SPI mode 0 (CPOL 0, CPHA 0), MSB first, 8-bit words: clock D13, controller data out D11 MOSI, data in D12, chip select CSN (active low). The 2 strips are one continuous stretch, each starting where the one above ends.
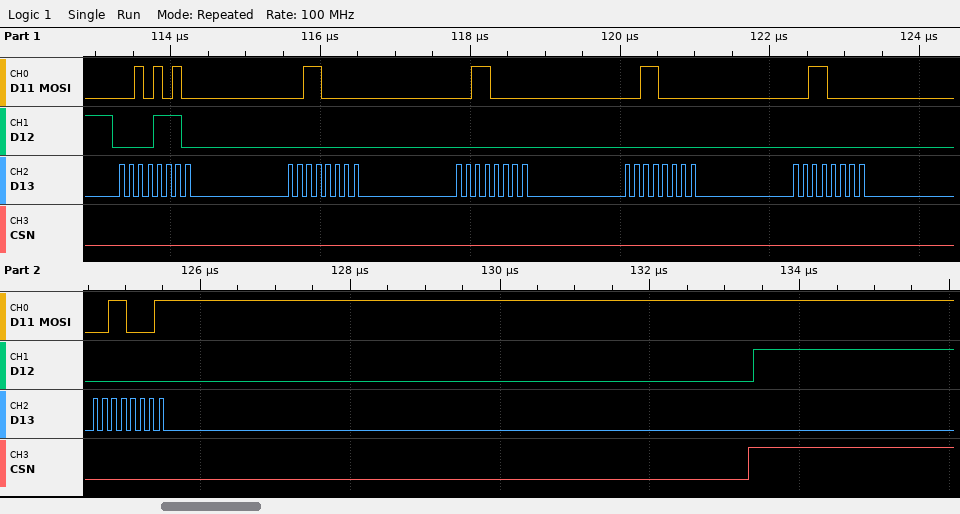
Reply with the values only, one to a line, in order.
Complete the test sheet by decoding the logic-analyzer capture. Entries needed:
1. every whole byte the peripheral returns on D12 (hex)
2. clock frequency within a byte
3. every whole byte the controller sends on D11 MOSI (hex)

0x0E 0x00 0x00 0x00 0x00 0x00
8 MHz
0x2A 0x30 0x30 0x30 0x30 0x31
